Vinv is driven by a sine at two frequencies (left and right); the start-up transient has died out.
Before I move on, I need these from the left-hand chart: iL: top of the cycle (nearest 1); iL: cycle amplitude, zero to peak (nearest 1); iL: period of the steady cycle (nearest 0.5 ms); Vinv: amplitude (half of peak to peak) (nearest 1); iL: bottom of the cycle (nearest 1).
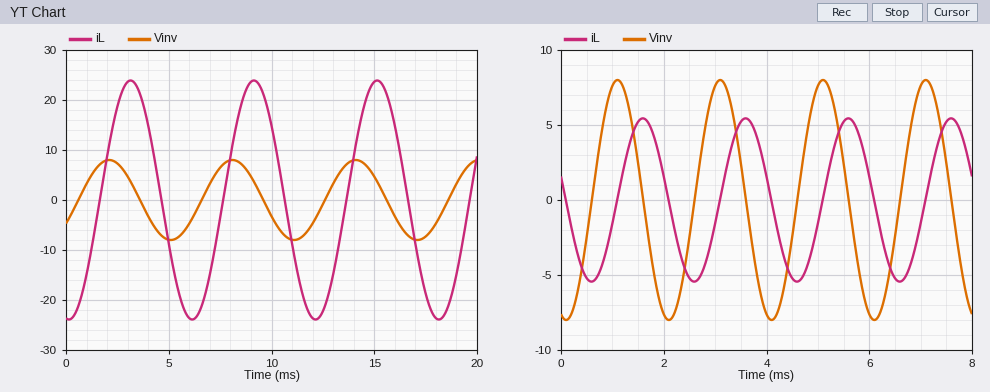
24
24
6.0 ms
8
-24
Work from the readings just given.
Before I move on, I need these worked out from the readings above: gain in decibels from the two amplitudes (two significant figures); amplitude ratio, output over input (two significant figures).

9.5 dB
3.0
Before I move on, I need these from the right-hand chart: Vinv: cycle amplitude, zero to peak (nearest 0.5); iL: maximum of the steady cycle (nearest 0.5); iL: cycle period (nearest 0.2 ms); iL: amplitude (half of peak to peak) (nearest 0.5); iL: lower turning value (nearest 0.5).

8.0
5.5
2.0 ms
5.5
-5.5
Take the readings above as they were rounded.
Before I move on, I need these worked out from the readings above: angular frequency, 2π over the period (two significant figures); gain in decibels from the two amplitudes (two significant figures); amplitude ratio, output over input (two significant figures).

3.1 rad/ms
-3.3 dB
0.69
